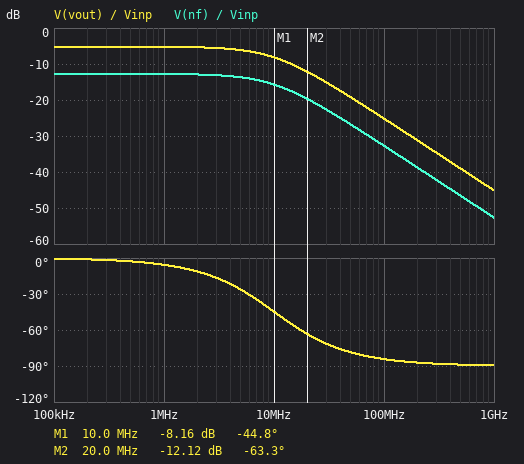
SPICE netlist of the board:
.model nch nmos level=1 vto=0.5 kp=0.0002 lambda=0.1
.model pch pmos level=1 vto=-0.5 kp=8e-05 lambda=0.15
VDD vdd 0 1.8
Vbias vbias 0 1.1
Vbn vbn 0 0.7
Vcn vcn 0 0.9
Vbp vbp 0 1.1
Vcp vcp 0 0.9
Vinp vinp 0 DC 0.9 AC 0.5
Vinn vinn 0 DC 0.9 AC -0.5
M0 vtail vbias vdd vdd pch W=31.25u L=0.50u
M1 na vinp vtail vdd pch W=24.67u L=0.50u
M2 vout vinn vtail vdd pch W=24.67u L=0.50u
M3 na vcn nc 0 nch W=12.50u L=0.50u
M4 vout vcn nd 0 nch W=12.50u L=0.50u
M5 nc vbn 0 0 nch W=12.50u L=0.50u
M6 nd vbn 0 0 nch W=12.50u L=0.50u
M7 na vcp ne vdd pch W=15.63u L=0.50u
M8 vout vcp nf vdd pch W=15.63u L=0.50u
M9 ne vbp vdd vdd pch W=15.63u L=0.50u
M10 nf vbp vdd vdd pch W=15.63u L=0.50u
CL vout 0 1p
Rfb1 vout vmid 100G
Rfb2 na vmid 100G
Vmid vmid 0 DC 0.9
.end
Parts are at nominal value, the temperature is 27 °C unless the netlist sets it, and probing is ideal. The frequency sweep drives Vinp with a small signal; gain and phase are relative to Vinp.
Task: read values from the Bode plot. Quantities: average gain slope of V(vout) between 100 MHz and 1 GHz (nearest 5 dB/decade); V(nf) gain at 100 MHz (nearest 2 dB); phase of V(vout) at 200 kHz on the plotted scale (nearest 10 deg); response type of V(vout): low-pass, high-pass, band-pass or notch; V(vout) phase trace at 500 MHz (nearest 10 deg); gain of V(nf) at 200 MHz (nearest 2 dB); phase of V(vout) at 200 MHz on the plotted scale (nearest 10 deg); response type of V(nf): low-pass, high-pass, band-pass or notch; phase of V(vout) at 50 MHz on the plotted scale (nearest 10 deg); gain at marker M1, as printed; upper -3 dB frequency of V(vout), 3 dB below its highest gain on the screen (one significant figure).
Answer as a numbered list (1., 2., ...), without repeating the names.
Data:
1. -20 dB/decade
2. -32 dB
3. 0 deg
4. low-pass
5. -90 deg
6. -38 dB
7. -90 deg
8. low-pass
9. -80 deg
10. -8.16 dB
11. 10 MHz
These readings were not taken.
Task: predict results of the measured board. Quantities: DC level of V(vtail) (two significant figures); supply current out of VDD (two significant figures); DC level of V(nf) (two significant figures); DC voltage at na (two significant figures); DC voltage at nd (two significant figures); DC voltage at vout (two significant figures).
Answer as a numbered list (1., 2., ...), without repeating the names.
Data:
1. 1.6 V
2. 200 µA
3. 1.6 V
4. 1.5 V
5. 210 mV
6. 1.5 V
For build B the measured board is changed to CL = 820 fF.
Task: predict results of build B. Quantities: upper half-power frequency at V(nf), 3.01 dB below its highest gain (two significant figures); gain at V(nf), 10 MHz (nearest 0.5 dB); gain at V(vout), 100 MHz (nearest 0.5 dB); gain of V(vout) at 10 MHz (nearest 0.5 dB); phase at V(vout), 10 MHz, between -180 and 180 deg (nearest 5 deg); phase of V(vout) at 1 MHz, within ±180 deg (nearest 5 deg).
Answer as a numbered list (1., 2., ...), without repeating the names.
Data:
1. 12 MHz
2. -15.0 dB
3. -23.5 dB
4. -7.5 dB
5. -40 deg
6. -5 deg
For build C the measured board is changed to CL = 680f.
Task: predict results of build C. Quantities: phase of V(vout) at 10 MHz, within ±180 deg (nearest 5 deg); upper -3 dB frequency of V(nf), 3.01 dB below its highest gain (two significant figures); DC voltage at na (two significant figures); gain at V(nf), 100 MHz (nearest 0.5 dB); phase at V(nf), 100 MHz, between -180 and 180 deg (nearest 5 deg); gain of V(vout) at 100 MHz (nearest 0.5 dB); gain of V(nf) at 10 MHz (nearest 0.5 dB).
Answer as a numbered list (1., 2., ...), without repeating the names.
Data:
1. -35 deg
2. 15 MHz
3. 1.5 V
4. -29.5 dB
5. -80 deg
6. -22.0 dB
7. -14.5 dB
